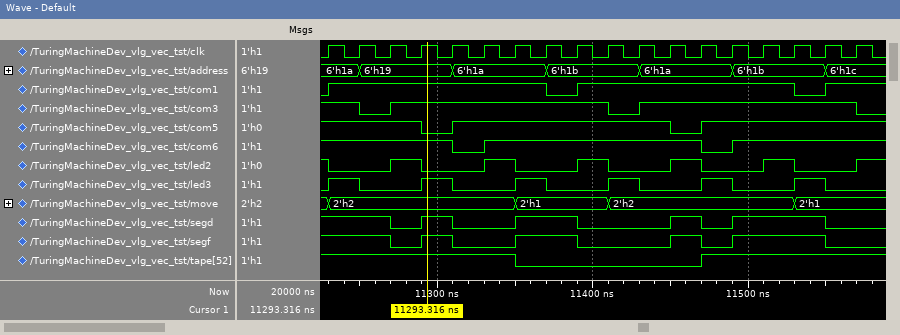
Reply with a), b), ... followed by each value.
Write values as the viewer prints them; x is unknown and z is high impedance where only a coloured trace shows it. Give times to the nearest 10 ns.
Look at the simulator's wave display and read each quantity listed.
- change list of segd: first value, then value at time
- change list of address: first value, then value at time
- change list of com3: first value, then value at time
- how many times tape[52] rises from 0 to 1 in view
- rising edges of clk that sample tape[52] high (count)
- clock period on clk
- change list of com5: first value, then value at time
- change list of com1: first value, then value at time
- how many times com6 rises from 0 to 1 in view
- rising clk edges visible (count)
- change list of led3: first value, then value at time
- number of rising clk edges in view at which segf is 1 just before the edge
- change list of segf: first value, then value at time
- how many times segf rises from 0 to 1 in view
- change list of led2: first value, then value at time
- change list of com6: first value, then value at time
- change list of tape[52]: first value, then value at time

a) 1, 0 at 11270 ns, 1 at 11290 ns, 0 at 11310 ns, 1 at 11350 ns, 0 at 11390 ns, 1 at 11450 ns, 0 at 11470 ns, 1 at 11490 ns, 0 at 11550 ns
b) 6'h1a, 6'h19 at 11250 ns, 6'h1a at 11310 ns, 6'h1b at 11370 ns, 6'h1a at 11430 ns, 6'h1b at 11490 ns, 6'h1c at 11550 ns
c) 1, 0 at 11250 ns, 1 at 11270 ns, 0 at 11410 ns, 1 at 11430 ns, 0 at 11570 ns
d) 1
e) 12
f) 20 ns
g) 1, 0 at 11290 ns, 1 at 11310 ns, 0 at 11450 ns, 1 at 11470 ns
h) 0, 1 at 11230 ns, 0 at 11370 ns, 1 at 11390 ns, 0 at 11530 ns, 1 at 11550 ns
i) 2
j) 18
k) 0, 1 at 11230 ns, 0 at 11250 ns, 1 at 11290 ns, 0 at 11310 ns, 1 at 11350 ns, 0 at 11370 ns, 1 at 11410 ns, 0 at 11430 ns, 1 at 11470 ns, 0 at 11490 ns, 1 at 11530 ns, 0 at 11550 ns
l) 10
m) 1, 0 at 11270 ns, 1 at 11290 ns, 0 at 11310 ns, 1 at 11350 ns, 0 at 11390 ns, 1 at 11450 ns, 0 at 11470 ns, 1 at 11490 ns, 0 at 11550 ns
n) 4
o) 1, 0 at 11230 ns, 1 at 11270 ns, 0 at 11290 ns, 1 at 11330 ns, 0 at 11350 ns, 1 at 11390 ns, 0 at 11410 ns, 1 at 11450 ns, 0 at 11470 ns, 1 at 11510 ns, 0 at 11530 ns, 1 at 11570 ns
p) 1, 0 at 11310 ns, 1 at 11330 ns, 0 at 11470 ns, 1 at 11490 ns
q) 1, 0 at 11350 ns, 1 at 11470 ns
